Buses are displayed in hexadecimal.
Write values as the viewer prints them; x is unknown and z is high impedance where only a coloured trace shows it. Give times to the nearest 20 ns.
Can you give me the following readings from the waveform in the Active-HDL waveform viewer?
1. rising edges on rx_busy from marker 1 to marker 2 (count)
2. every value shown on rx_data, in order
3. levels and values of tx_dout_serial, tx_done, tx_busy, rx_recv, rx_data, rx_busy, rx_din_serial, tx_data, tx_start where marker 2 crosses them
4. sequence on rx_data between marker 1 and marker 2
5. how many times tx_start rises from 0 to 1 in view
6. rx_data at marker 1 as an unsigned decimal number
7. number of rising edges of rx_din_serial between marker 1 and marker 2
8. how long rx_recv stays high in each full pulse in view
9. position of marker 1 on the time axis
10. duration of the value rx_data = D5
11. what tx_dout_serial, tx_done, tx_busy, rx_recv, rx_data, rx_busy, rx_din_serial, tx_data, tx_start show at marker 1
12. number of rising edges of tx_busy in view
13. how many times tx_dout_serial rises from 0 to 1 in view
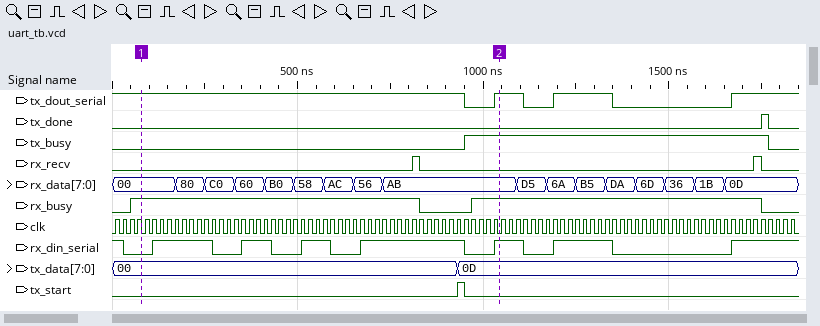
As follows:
1
00, 80, C0, 60, B0, 58, AC, 56, AB, D5, 6A, B5, DA, 6D, 36, 1B, 0D
tx_dout_serial=1, tx_done=0, tx_busy=1, rx_recv=0, rx_data=AB, rx_busy=1, rx_din_serial=1, tx_data=0D, tx_start=0
00, 80, C0, 60, B0, 58, AC, 56, AB
1
0
5
20 ns, 20 ns
80 ns
80 ns
tx_dout_serial=1, tx_done=0, tx_busy=0, rx_recv=0, rx_data=00, rx_busy=1, rx_din_serial=0, tx_data=00, tx_start=0
1
3
